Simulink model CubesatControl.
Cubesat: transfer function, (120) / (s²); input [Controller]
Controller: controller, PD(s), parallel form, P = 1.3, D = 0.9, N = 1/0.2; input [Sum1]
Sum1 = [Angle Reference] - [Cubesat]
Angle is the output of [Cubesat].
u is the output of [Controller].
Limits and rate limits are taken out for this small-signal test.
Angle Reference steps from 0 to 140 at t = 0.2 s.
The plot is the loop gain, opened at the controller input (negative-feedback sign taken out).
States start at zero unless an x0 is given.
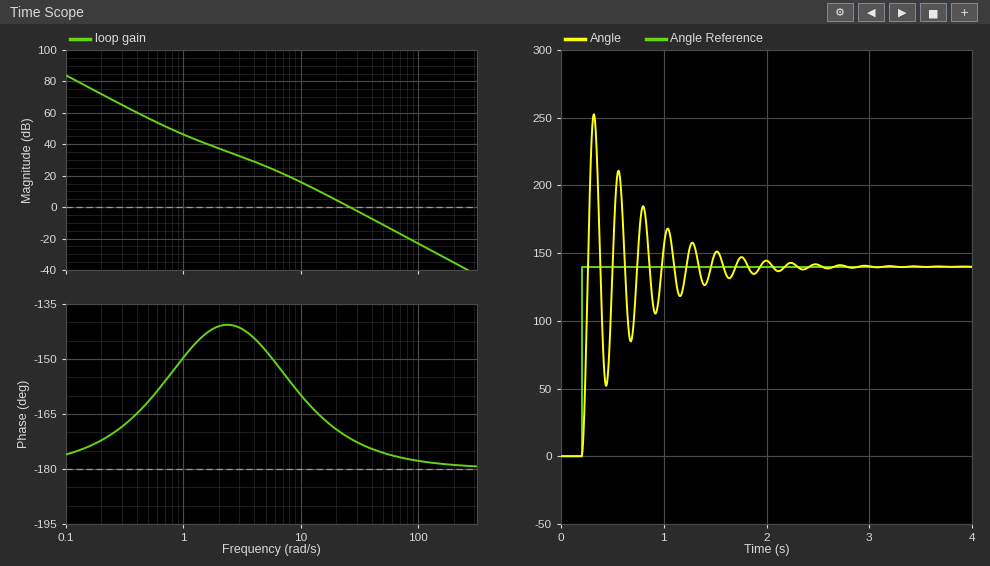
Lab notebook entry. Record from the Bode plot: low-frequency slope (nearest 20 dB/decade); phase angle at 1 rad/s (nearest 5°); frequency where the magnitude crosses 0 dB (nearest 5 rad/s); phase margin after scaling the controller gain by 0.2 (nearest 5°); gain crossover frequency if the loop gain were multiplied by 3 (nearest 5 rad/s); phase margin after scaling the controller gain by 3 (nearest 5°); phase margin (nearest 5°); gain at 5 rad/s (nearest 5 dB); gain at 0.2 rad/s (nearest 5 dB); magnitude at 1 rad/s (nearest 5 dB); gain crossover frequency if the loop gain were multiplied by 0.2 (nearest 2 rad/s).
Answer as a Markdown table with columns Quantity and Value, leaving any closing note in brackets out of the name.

| Quantity | Value |
|---|---|
| low-frequency slope | -40 dB/decade |
| phase angle at 1 rad/s | -150° |
| frequency where the magnitude crosses 0 dB | 25 rad/s |
| phase margin after scaling the controller gain by 0.2 | 20° |
| gain crossover frequency if the loop gain were multiplied by 3 | 45 rad/s |
| phase margin after scaling the controller gain by 3 | 5° |
| phase margin | 10° |
| gain at 5 rad/s | 25 dB |
| gain at 0.2 rad/s | 70 dB |
| magnitude at 1 rad/s | 45 dB |
| gain crossover frequency if the loop gain were multiplied by 0.2 | 12 rad/s |
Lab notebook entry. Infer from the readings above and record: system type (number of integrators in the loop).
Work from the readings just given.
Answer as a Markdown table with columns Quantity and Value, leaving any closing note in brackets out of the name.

| Quantity | Value |
|---|---|
| system type | 2 |
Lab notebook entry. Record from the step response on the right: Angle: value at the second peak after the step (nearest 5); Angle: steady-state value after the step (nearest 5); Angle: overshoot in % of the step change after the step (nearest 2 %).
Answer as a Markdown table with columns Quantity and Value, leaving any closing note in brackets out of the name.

| Quantity | Value |
|---|---|
| Angle: value at the second peak after the step | 210 |
| Angle: steady-state value after the step | 140 |
| Angle: overshoot in % of the step change after the step | 80 % |
